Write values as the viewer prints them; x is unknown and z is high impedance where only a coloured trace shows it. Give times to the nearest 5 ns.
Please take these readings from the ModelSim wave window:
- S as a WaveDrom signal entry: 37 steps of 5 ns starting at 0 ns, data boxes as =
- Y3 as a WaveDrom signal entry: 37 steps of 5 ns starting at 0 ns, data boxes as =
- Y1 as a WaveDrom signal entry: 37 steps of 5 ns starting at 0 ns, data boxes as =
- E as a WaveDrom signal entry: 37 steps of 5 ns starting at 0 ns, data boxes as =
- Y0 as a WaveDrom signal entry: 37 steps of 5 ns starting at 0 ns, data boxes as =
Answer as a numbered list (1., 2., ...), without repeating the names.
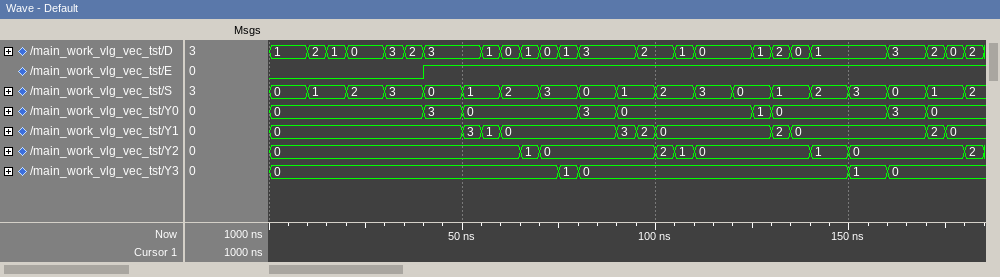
1. {name: 'S', wave: '=.=.=.=.=.=.=.=.=.=.=.=.=.=.=.=.=.=.=', data: '0 1 2 3 0 1 2 3 0 1 2 3 0 1 2 3 0 1 2'}
2. {name: 'Y3', wave: '=..............==.............=.=....', data: '0 1 0 1 0'}
3. {name: 'Y1', wave: '=.........===.....===.....==......==.', data: '0 3 1 0 3 2 0 2 0 2 0'}
4. {name: 'E', wave: '0.......1............................'}
5. {name: 'Y0', wave: '=.......=.=.....=.=......==.....=.=..', data: '0 3 0 3 0 1 0 3 0'}
